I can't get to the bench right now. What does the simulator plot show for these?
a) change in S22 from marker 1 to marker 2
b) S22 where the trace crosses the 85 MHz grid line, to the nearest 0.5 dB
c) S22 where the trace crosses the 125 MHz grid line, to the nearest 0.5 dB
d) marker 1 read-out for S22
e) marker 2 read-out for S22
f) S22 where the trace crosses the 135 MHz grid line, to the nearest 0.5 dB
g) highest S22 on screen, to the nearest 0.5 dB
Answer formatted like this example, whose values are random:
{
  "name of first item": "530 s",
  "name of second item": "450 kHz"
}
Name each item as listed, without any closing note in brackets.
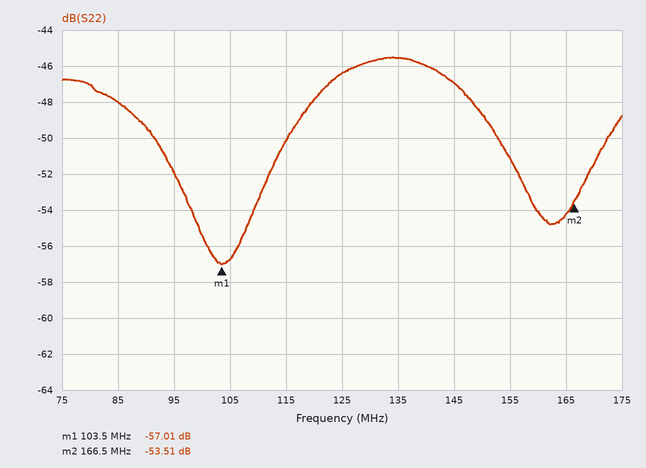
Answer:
{
  "change in S22 from marker 1 to marker 2": "3.50 dB",
  "S22 where the trace crosses the 85 MHz grid line, to the nearest 0.5 dB": "-48.0 dB",
  "S22 where the trace crosses the 125 MHz grid line, to the nearest 0.5 dB": "-46.5 dB",
  "marker 1 read-out for S22": "-57.01 dB",
  "marker 2 read-out for S22": "-53.51 dB",
  "S22 where the trace crosses the 135 MHz grid line, to the nearest 0.5 dB": "-45.5 dB",
  "highest S22 on screen, to the nearest 0.5 dB": "-45.5 dB"
}
